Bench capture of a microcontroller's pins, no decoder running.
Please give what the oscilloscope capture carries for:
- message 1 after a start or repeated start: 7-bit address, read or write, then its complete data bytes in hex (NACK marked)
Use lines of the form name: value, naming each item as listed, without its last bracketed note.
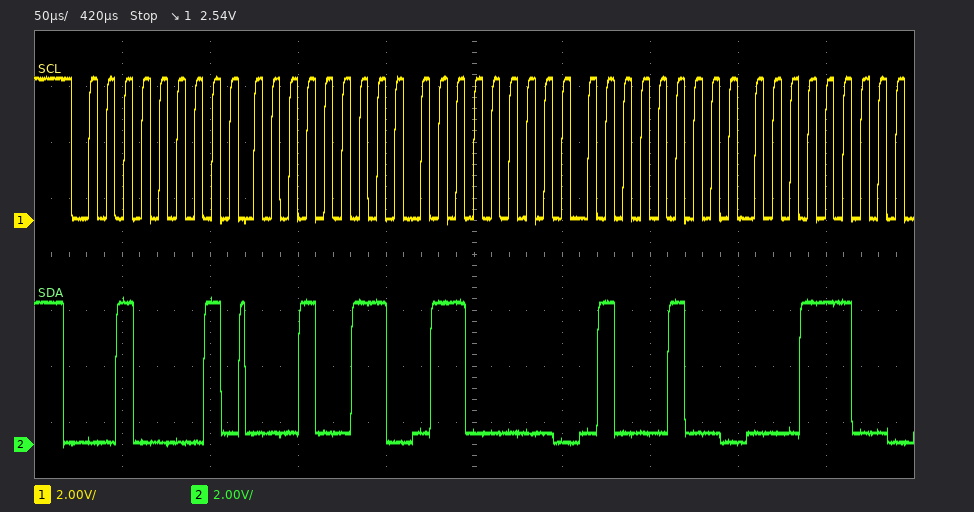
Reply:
message 1 after a start or repeated start: 7-bit address, read or write, then its complete data bytes in hex: 0x10 read: 13 60 44 1C
